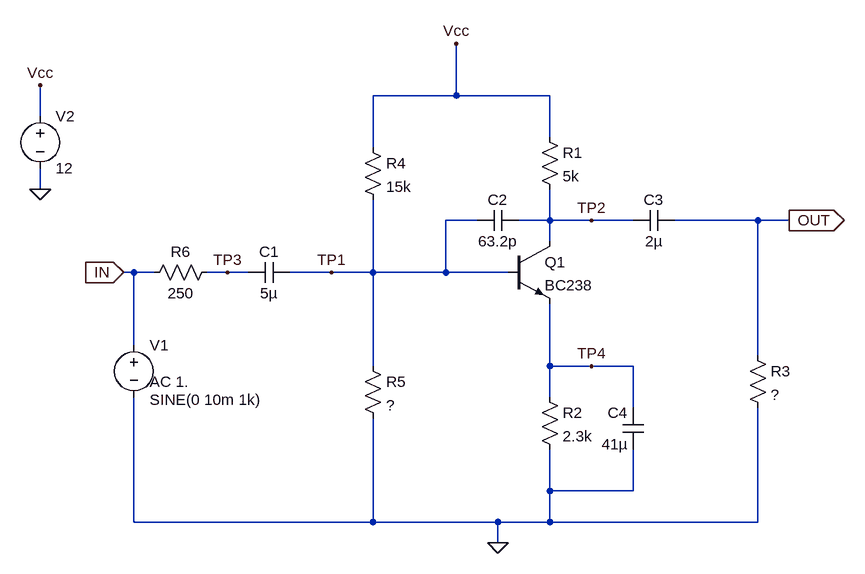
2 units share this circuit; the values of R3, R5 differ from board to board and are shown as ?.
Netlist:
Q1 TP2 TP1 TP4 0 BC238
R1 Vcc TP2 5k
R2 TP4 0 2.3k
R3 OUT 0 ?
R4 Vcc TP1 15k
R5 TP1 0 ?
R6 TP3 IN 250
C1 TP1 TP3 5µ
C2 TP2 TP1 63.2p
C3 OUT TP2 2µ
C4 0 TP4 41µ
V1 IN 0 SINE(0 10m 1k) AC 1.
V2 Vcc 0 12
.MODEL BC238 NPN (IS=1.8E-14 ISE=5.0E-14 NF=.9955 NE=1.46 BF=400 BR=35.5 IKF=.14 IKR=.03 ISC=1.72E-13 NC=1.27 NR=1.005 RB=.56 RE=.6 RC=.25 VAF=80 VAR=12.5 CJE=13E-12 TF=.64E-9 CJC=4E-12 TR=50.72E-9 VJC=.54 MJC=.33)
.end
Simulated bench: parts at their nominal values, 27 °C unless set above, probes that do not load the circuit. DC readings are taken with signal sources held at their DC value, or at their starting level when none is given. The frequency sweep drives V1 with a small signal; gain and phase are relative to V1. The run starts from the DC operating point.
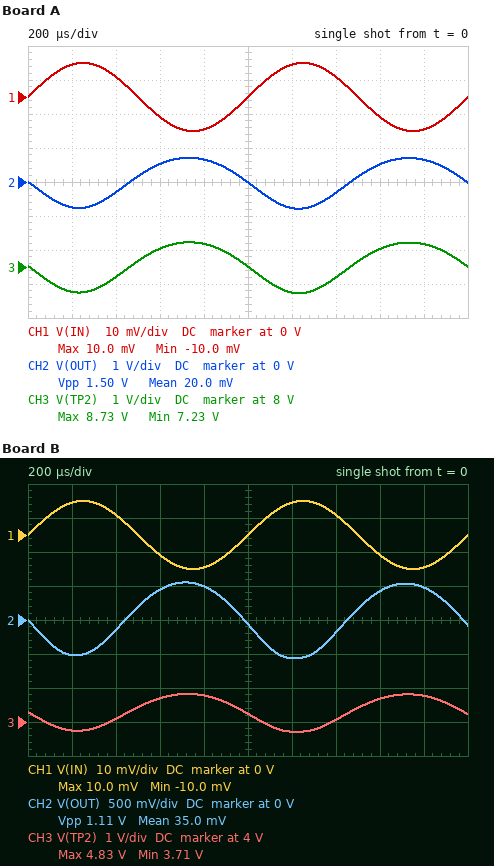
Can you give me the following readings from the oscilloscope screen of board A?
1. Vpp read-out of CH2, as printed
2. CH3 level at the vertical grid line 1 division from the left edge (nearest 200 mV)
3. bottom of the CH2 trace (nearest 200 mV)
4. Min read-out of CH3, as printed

1.50 V
7.2 V
-800 mV
7.23 V
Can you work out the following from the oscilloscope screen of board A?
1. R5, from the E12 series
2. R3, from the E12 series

3.9 kΩ
6.8 kΩ
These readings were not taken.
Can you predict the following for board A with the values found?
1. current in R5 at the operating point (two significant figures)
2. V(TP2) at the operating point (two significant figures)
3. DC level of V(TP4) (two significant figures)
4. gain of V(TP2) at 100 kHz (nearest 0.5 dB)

630 µA
8.0 V
1.8 V
35.0 dB
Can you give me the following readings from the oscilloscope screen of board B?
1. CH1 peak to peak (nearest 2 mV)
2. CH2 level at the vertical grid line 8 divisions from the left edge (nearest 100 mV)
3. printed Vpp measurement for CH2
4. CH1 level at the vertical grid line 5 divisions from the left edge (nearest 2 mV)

20 mV
400 mV
1.11 V
0 V
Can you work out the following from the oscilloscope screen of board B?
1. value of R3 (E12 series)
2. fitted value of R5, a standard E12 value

1.5 kΩ
8.2 kΩ
